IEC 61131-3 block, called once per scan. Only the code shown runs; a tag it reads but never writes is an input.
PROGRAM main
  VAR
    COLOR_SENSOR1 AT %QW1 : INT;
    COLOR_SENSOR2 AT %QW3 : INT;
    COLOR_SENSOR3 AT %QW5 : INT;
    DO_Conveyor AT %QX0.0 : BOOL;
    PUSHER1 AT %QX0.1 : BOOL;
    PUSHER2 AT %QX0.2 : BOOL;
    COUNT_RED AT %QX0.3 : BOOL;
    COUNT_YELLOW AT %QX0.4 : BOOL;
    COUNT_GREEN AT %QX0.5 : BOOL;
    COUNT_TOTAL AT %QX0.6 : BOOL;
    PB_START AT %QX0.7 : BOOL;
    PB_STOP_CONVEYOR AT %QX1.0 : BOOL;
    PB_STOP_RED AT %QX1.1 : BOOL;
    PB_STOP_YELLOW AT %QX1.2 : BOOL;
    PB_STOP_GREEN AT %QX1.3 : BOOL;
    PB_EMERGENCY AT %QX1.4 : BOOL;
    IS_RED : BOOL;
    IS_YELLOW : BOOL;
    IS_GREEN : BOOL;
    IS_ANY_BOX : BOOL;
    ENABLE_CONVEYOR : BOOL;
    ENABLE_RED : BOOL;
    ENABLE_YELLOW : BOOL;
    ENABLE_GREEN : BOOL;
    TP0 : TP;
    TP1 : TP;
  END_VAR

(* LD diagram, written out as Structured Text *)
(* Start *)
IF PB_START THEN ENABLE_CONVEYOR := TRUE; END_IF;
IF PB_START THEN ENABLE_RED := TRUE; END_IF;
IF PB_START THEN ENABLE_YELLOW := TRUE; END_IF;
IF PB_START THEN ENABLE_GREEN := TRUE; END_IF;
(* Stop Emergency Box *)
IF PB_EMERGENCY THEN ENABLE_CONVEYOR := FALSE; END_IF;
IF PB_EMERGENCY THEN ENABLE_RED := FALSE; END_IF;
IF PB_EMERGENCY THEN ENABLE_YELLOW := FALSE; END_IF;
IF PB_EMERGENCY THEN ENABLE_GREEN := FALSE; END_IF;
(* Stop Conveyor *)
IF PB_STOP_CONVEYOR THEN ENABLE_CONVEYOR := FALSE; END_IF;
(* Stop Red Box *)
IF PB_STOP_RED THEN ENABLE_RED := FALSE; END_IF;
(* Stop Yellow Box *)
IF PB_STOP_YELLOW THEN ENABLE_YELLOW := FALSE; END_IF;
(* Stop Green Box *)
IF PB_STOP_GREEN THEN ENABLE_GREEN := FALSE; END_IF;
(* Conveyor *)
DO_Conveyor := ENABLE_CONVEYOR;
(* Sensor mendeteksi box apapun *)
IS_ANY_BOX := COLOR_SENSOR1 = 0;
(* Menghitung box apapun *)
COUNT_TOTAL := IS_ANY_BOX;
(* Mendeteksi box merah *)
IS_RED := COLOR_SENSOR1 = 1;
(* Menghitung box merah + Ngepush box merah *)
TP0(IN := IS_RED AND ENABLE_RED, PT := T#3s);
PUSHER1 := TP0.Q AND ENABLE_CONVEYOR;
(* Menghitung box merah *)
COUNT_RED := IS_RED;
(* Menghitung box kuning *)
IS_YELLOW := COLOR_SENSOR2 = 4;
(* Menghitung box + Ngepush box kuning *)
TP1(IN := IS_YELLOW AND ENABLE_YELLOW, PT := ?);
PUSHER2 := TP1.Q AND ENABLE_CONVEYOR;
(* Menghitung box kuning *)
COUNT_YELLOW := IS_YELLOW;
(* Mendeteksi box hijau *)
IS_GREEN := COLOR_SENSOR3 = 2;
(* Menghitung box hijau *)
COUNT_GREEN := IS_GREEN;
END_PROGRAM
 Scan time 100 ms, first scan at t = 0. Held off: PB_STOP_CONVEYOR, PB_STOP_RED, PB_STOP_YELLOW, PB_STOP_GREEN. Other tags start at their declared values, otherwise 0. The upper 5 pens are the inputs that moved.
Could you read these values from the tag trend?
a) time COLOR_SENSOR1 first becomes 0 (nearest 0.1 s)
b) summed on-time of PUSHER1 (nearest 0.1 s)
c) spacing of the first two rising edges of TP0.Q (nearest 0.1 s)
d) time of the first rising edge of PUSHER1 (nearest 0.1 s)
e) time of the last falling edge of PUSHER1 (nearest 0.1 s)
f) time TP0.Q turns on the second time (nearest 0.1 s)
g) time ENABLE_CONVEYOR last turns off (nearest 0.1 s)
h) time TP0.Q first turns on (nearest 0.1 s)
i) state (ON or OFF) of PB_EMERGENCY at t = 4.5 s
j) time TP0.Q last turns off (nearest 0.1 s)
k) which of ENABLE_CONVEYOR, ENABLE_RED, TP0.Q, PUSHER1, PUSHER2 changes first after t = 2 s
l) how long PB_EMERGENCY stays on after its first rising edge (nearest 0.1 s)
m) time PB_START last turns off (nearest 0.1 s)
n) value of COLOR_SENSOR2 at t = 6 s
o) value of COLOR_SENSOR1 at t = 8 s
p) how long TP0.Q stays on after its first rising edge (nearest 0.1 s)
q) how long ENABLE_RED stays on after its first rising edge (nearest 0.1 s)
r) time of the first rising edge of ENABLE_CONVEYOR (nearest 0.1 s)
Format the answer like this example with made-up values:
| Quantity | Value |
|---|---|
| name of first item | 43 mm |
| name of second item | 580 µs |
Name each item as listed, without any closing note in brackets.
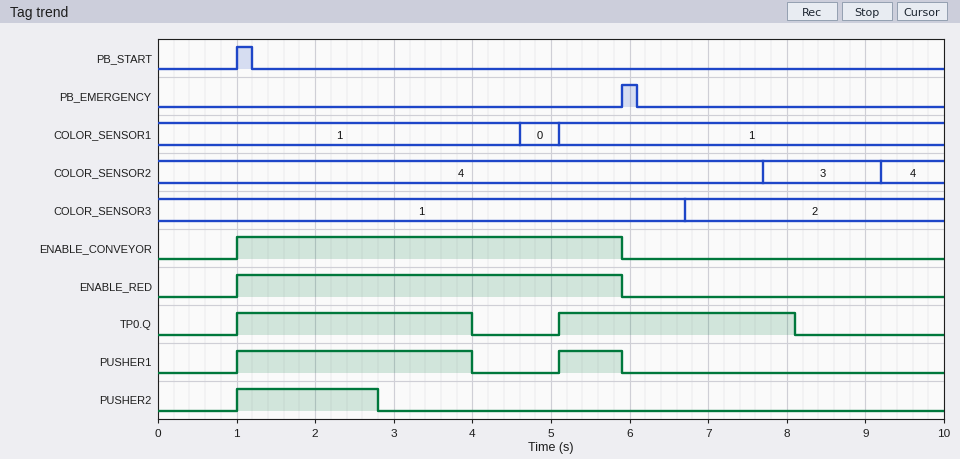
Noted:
| Quantity | Value |
|---|---|
| time COLOR_SENSOR1 first becomes 0 | 4.6 s |
| summed on-time of PUSHER1 | 3.8 s |
| spacing of the first two rising edges of TP0.Q | 4.1 s |
| time of the first rising edge of PUSHER1 | 1.0 s |
| time of the last falling edge of PUSHER1 | 5.9 s |
| time TP0.Q turns on the second time | 5.1 s |
| time ENABLE_CONVEYOR last turns off | 5.9 s |
| time TP0.Q first turns on | 1.0 s |
| state (ON or OFF) of PB_EMERGENCY at t = 4.5 s | OFF |
| time TP0.Q last turns off | 8.1 s |
| which of ENABLE_CONVEYOR, ENABLE_RED, TP0.Q, PUSHER1, PUSHER2 changes first after t = 2 s | PUSHER2 |
| how long PB_EMERGENCY stays on after its first rising edge | 0.2 s |
| time PB_START last turns off | 1.2 s |
| value of COLOR_SENSOR2 at t = 6 s | 4 |
| value of COLOR_SENSOR1 at t = 8 s | 1 |
| how long TP0.Q stays on after its first rising edge | 3.0 s |
| how long ENABLE_RED stays on after its first rising edge | 4.9 s |
| time of the first rising edge of ENABLE_CONVEYOR | 1.0 s |
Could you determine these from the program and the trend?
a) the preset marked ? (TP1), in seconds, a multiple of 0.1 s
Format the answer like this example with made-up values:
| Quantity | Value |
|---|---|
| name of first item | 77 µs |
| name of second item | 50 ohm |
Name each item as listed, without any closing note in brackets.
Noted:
| Quantity | Value |
|---|---|
| the preset marked ? (TP1), in seconds, a multiple of 0.1 s | 1.8 s |
